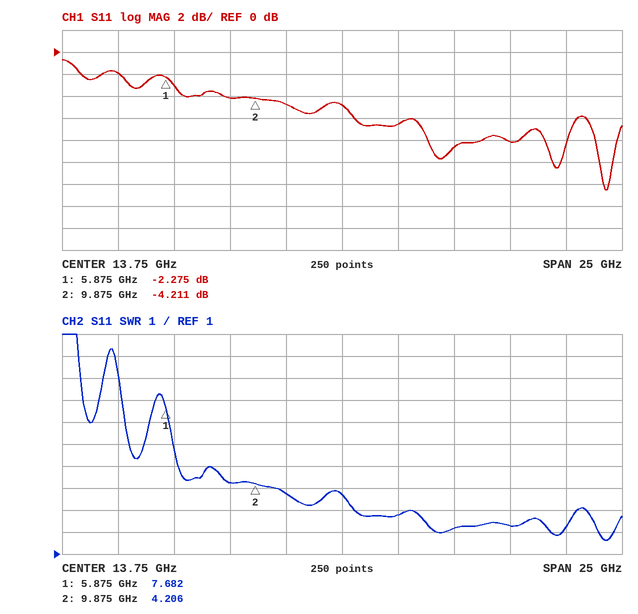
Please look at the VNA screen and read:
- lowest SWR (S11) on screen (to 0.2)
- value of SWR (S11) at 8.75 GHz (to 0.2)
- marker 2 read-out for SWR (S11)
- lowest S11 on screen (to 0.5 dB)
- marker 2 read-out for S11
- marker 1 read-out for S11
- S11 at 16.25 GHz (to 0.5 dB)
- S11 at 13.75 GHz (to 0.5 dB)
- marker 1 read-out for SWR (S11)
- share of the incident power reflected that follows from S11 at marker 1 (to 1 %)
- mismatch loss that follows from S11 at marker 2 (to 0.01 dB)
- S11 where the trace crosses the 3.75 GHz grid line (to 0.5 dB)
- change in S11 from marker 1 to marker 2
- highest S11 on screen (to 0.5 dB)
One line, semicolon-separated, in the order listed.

1.6; 4.2; 4.206; -12.5 dB; -4.211 dB; -2.275 dB; -6.5 dB; -5.0 dB; 7.682; 59 %; 2.07 dB; -2.0 dB; -1.936 dB; -0.5 dB
